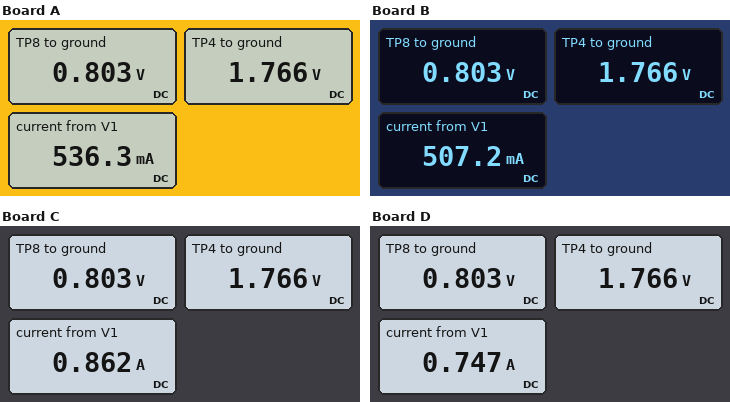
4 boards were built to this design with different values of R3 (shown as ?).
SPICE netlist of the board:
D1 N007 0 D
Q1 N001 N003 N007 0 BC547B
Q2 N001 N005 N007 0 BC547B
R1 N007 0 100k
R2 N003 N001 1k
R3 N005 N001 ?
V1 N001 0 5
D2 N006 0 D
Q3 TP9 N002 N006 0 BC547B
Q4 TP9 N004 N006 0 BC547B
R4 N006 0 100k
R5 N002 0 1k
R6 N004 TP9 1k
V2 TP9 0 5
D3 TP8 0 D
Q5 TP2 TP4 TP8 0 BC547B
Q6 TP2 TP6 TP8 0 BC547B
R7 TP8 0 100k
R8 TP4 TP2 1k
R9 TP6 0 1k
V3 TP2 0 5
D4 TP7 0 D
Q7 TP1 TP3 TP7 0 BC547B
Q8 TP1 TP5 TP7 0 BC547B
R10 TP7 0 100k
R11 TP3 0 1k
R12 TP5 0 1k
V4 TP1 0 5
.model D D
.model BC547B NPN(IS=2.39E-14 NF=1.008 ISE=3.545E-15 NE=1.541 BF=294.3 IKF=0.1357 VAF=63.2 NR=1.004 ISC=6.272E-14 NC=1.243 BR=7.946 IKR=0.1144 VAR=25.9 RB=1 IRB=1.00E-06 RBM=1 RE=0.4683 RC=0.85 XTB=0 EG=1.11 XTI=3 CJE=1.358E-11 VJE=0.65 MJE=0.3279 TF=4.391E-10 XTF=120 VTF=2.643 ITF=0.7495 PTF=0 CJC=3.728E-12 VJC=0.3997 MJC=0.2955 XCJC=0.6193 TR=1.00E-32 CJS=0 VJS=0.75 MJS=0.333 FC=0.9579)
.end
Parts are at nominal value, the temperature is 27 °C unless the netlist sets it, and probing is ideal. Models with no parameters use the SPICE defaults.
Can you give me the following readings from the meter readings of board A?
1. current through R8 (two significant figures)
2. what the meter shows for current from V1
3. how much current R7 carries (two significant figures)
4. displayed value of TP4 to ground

3.2 mA
536.3 mA
8.0 µA
1.766 V
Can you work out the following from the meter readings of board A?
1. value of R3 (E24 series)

1.6 kΩ
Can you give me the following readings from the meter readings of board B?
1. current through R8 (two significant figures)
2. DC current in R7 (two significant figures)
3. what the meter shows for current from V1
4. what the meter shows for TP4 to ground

3.2 mA
8.0 µA
507.2 mA
1.766 V
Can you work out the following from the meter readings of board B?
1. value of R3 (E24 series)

2 kΩ
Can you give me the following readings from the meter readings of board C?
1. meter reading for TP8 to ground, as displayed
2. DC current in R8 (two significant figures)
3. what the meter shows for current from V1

0.803 V
3.2 mA
0.862 A
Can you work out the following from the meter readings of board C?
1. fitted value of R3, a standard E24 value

330 Ω
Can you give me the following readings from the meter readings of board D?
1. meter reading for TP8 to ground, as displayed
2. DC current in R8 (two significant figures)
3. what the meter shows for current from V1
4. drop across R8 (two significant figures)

0.803 V
3.2 mA
0.747 A
3.2 V
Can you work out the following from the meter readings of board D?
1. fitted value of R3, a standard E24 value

510 Ω
